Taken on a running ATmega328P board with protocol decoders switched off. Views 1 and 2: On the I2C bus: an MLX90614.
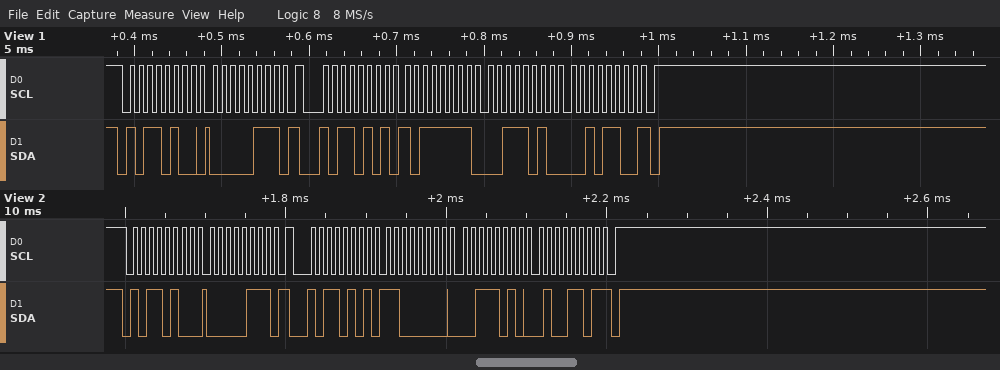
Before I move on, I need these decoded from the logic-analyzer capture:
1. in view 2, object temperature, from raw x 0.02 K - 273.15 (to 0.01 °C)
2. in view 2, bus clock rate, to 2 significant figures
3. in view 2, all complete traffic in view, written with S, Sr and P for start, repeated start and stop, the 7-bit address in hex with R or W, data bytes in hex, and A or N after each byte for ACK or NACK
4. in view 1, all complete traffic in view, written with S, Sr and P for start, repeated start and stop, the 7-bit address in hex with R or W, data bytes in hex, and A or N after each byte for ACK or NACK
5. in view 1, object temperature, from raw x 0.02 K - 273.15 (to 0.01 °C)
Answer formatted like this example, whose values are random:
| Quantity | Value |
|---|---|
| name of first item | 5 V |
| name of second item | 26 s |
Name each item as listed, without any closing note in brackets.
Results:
| Quantity | Value |
|---|---|
| in view 2, object temperature, from raw x 0.02 K - 273.15 | 27.65 °C |
| in view 2, bus clock rate, to 2 significant figures | 100 kHz |
| in view 2, all complete traffic in view, written with S, Sr and P for start, repeated start and stop, the 7-bit address in hex with R or W, data bytes in hex, and A or N after each byte for ACK or NACK | S 5AW A 07 A Sr 5AR A C0 A 3A A 4D N P |
| in view 1, all complete traffic in view, written with S, Sr and P for start, repeated start and stop, the 7-bit address in hex with R or W, data bytes in hex, and A or N after each byte for ACK or NACK | S 5AW A 07 A Sr 5AR A BF A 3A A 2C N P |
| in view 1, object temperature, from raw x 0.02 K - 273.15 | 27.63 °C |
